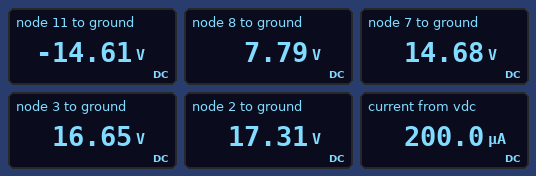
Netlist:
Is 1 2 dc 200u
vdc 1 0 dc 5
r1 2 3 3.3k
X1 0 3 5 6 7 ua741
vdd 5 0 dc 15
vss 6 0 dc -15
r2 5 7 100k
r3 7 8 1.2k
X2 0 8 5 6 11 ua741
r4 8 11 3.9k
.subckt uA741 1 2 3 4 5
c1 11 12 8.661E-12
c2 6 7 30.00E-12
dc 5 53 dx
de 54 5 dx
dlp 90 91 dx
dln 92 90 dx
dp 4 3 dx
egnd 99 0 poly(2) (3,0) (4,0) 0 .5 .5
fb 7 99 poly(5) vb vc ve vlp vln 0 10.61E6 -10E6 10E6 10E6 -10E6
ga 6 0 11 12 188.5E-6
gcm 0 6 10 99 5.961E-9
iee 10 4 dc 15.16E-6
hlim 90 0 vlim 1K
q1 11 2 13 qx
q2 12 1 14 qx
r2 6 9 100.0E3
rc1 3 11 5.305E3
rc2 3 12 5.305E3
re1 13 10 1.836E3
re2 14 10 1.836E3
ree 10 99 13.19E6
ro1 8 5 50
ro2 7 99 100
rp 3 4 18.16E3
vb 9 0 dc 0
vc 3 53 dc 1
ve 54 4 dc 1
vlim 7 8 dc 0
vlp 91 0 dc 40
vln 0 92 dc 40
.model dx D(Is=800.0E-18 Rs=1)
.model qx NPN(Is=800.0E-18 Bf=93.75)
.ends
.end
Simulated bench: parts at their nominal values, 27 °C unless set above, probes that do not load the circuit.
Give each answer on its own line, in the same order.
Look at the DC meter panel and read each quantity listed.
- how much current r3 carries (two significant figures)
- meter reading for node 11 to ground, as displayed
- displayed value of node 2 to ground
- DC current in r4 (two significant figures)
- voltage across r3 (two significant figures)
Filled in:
5.7 mA
-14.61 V
17.31 V
5.7 mA
6.9 V
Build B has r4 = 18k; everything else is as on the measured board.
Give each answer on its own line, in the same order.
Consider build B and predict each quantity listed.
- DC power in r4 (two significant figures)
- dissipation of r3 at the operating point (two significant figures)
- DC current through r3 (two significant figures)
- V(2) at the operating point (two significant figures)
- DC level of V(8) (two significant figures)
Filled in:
42 mW
2.8 mW
1.5 mA
17 V
13 V
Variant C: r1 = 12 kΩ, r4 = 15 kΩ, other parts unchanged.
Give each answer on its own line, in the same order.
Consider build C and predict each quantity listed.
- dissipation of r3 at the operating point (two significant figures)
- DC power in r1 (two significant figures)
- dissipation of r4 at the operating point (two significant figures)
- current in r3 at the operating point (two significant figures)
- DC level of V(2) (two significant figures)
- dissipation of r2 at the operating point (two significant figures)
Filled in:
3.9 mW
480 µW
49 mW
1.8 mA
19 V
1.0 µW
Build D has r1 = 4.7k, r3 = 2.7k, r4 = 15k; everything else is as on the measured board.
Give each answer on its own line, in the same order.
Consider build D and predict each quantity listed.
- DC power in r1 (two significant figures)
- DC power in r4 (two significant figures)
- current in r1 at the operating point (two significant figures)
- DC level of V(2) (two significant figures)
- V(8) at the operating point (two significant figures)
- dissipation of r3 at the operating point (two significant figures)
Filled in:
190 µW
41 mW
200 µA
18 V
10 V
7.4 mW
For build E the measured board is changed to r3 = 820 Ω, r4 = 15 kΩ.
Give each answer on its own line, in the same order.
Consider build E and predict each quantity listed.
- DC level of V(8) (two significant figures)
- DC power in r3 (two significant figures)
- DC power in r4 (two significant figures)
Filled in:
13 V
2.8 mW
51 mW
